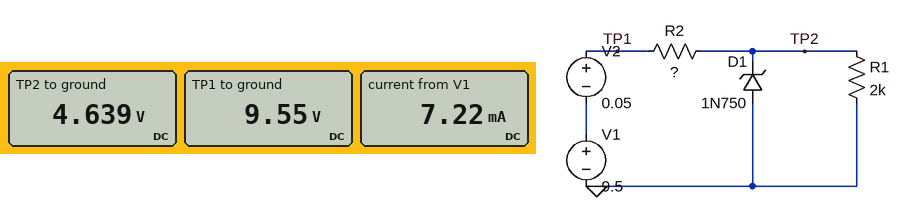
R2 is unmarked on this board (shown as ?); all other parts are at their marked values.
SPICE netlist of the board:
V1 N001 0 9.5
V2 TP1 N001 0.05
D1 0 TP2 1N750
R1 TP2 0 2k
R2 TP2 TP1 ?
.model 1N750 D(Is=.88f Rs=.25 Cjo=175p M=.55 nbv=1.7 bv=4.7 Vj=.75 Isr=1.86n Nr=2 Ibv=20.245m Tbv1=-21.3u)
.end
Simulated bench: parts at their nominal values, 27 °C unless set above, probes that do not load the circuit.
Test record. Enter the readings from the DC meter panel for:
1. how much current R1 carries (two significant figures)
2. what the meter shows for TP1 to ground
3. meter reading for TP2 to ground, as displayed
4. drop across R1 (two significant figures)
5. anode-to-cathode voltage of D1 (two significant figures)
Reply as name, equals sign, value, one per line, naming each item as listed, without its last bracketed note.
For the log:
how much current R1 carries = 2.3 mA
what the meter shows for TP1 to ground = 9.55 V
meter reading for TP2 to ground, as displayed = 4.639 V
drop across R1 = 4.6 V
anode-to-cathode voltage of D1 = -4.6 V
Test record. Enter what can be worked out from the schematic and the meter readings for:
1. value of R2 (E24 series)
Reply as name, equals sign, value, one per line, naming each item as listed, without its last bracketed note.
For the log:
value of R2 = 680 Ω
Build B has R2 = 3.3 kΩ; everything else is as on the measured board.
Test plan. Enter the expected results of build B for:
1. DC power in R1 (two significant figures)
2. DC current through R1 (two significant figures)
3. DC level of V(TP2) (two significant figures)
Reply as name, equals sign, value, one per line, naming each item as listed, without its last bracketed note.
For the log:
DC power in R1 = 6.5 mW
DC current through R1 = 1.8 mA
DC level of V(TP2) = 3.6 V
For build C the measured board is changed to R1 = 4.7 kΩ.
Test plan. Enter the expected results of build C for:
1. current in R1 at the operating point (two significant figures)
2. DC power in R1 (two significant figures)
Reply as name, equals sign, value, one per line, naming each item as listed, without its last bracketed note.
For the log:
current in R1 at the operating point = 990 µA
DC power in R1 = 4.6 mW
